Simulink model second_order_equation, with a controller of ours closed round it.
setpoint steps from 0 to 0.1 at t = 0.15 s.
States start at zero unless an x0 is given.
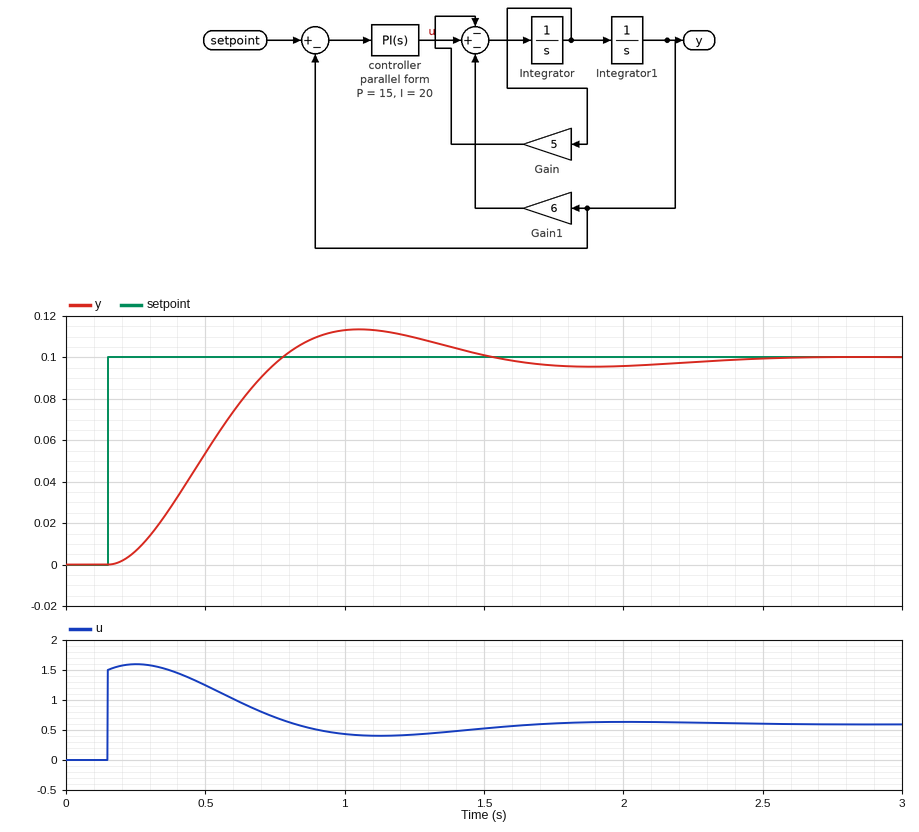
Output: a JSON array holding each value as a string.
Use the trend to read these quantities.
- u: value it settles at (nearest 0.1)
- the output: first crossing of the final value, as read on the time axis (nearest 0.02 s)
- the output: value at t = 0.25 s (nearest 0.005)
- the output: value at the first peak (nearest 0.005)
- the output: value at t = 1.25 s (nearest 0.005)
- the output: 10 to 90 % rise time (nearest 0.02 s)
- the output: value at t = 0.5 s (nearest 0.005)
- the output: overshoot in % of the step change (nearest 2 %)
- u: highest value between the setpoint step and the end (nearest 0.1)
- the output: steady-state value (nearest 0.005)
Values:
["0.6", "0.78 s", "0.005", "0.115", "0.110", "0.42 s", "0.055", "14 %", "1.6", "0.100"]
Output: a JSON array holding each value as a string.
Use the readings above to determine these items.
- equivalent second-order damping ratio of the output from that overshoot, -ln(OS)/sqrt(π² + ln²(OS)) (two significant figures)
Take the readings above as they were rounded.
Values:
["0.53"]
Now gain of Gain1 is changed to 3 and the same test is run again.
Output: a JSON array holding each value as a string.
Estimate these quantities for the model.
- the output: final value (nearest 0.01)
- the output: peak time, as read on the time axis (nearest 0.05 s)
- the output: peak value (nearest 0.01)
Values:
["0.10", "1.10 s", "0.13"]
